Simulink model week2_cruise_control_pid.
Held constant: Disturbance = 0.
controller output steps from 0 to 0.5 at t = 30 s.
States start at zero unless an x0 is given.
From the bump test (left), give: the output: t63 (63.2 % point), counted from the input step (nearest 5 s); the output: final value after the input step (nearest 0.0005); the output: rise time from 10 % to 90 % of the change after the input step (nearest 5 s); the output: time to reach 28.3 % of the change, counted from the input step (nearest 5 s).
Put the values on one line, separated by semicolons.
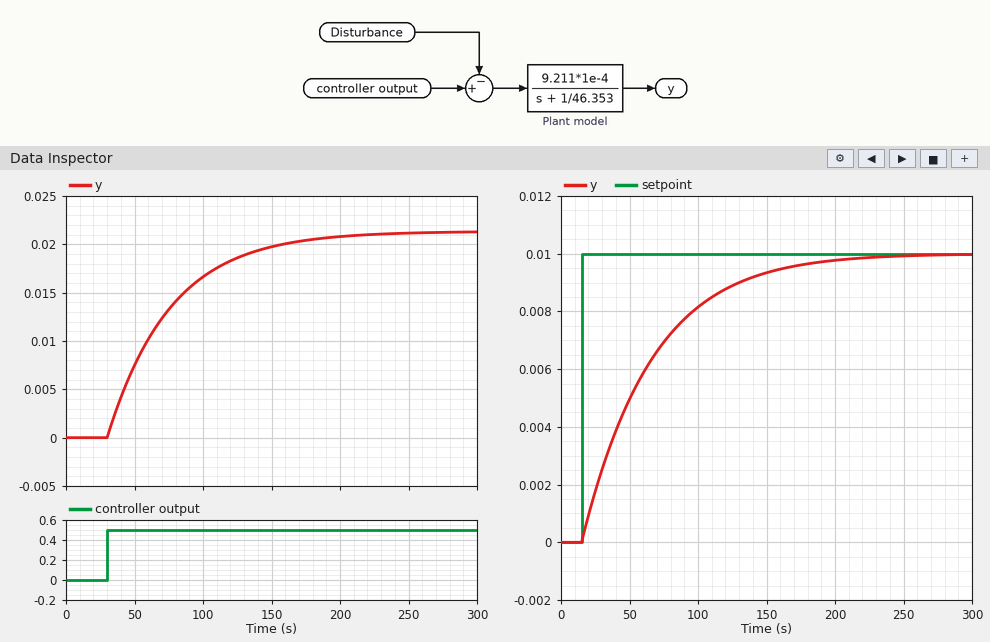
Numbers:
45 s; 0.0215; 100 s; 15 s
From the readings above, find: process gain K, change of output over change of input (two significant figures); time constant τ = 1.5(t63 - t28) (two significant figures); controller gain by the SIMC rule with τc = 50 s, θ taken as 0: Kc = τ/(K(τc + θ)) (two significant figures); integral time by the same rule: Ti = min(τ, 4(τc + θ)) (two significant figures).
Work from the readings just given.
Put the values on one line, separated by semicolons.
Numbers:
0.043; 45 s; 21; 45 s
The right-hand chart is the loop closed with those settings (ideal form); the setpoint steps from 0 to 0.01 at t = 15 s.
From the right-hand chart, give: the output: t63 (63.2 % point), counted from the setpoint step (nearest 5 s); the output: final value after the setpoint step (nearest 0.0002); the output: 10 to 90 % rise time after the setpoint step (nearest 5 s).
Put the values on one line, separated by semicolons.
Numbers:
50 s; 0.0100; 110 s
